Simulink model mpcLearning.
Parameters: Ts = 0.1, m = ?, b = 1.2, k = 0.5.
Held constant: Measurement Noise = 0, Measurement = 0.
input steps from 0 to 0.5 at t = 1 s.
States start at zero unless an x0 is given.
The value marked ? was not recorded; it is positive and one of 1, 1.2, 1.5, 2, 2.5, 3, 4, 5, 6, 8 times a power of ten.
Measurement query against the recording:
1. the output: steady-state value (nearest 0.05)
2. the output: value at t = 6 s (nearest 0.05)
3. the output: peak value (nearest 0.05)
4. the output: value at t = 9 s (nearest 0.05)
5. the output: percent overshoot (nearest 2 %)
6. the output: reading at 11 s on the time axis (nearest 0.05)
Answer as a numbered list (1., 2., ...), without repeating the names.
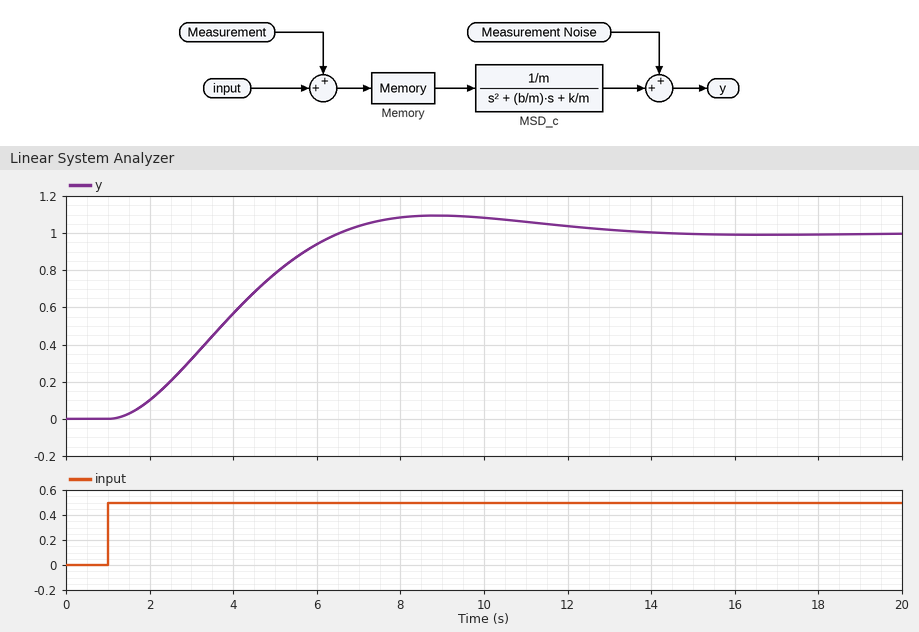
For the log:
1. 1.00
2. 0.95
3. 1.10
4. 1.10
5. 10 %
6. 1.05
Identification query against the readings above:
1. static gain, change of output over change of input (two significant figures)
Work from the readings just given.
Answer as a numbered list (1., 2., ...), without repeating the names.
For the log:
1. 2.0
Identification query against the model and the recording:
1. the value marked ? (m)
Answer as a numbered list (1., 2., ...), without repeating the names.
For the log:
1. 2
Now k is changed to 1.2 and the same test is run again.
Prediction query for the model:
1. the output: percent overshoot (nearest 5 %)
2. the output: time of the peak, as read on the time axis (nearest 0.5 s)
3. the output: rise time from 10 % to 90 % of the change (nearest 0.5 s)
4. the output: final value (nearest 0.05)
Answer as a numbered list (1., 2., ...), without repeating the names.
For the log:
1. 25 %
2. 5.5 s
3. 2.0 s
4. 0.40
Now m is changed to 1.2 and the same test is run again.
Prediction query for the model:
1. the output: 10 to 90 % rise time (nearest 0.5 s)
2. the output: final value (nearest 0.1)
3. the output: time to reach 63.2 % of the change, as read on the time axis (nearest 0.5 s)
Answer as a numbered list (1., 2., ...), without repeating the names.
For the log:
1. 3.5 s
2. 1.0
3. 4.0 s
